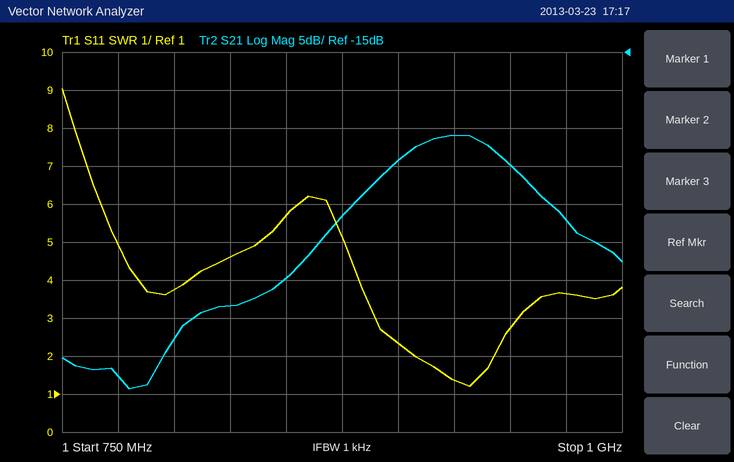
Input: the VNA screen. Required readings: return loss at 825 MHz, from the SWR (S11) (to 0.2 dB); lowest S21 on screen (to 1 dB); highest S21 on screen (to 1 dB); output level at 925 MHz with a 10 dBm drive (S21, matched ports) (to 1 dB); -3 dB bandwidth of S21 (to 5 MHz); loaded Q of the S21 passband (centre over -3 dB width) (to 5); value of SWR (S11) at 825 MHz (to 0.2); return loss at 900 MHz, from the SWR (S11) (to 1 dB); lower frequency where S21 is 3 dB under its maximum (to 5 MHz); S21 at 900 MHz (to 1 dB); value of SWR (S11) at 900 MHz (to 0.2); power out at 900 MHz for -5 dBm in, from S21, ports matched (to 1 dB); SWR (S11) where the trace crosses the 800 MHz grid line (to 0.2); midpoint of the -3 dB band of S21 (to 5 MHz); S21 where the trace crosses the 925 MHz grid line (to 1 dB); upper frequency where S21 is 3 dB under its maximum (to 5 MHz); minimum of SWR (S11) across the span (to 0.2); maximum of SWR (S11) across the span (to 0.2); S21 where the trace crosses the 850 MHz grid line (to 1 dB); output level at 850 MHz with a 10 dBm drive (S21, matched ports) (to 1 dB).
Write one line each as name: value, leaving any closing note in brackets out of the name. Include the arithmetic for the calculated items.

return loss at 825 MHz, from the SWR (S11): −20 log10((4.6 − 1)/(4.6 + 1)) ≈ 3.8 dB
lowest S21 on screen: -59 dB
highest S21 on screen: -26 dB
output level at 925 MHz with a 10 dBm drive (S21, matched ports): 10 dBm + (-26 dB) = -16 dBm
-3 dB bandwidth of S21: 945 MHz − 900 MHz = 45 MHz
loaded Q of the S21 passband (centre over -3 dB width): 922.5 MHz / 45 MHz ≈ 20
value of SWR (S11) at 825 MHz: 4.6
return loss at 900 MHz, from the SWR (S11): −20 log10((2.4 − 1)/(2.4 + 1)) ≈ 8 dB
lower frequency where S21 is 3 dB under its maximum: 900 MHz
S21 at 900 MHz: -29 dB
value of SWR (S11) at 900 MHz: 2.4
power out at 900 MHz for -5 dBm in, from S21, ports matched: -5 dBm + (-29 dB) = -34 dBm
SWR (S11) where the trace crosses the 800 MHz grid line: 3.8
midpoint of the -3 dB band of S21: 925 MHz
S21 where the trace crosses the 925 MHz grid line: -26 dB
upper frequency where S21 is 3 dB under its maximum: 945 MHz
minimum of SWR (S11) across the span: 1.2
maximum of SWR (S11) across the span: 9.0
S21 where the trace crosses the 850 MHz grid line: -45 dB
output level at 850 MHz with a 10 dBm drive (S21, matched ports): 10 dBm + (-45 dB) = -35 dBm
